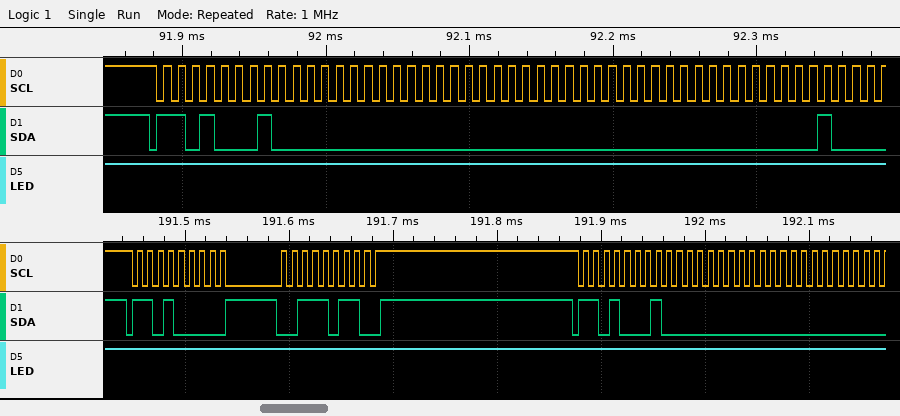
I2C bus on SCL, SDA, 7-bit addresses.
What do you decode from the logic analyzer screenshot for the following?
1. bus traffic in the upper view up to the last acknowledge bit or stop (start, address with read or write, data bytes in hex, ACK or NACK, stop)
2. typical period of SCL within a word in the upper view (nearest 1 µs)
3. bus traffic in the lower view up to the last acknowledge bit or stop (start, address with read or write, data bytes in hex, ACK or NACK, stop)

start, address 68 read ACK, 00 ACK, 00 ACK, 00 ACK, 00 ACK
10 µs
start, address 68 write ACK, 3B ACK, stop, start, address 68 read ACK, 00 ACK, 00 ACK
